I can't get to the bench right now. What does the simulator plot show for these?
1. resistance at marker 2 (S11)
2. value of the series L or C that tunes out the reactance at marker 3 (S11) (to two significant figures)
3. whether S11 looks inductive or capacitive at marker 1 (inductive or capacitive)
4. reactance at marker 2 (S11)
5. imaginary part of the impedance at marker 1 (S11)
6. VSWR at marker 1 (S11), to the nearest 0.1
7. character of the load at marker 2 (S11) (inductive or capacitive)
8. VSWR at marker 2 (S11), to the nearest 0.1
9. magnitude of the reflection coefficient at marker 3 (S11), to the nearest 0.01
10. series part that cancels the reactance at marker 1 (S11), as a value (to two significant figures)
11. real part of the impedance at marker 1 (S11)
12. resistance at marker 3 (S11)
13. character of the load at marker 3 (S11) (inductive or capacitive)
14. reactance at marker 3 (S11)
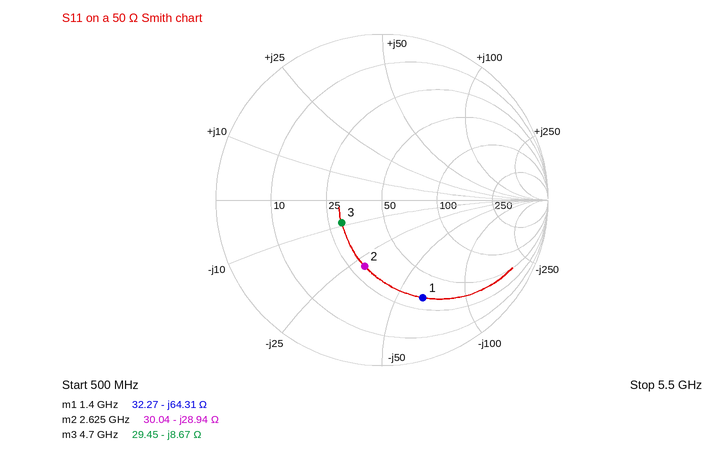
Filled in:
30.04 Ω
290 pH
capacitive
-28.94 Ω
-64.31 Ω
4.5
capacitive
2.4
0.28
7.3 nH
32.27 Ω
29.45 Ω
capacitive
-8.67 Ω
